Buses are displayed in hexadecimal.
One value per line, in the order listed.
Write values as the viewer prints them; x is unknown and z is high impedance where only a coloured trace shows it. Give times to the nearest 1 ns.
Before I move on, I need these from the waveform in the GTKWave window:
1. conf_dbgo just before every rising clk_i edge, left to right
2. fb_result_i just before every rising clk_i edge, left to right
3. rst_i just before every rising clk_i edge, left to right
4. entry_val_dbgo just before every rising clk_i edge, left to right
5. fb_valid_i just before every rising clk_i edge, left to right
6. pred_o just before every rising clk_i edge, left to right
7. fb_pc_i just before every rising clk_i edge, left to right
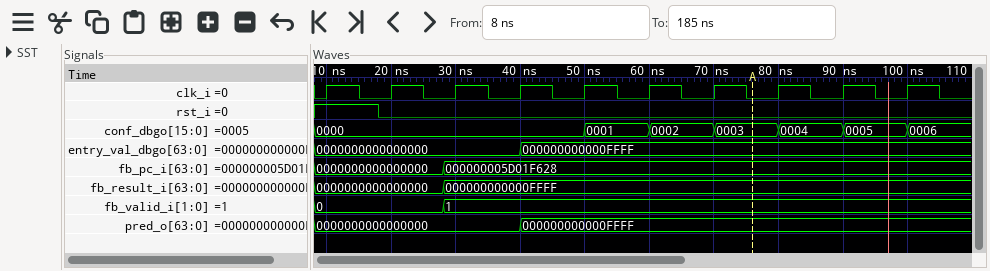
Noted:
0000, 0000, 0000, 0000, 0000, 0001, 0002, 0003, 0004, 0005
0000000000000000, 0000000000000000, 000000000000FFFF, 000000000000FFFF, 000000000000FFFF, 000000000000FFFF, 000000000000FFFF, 000000000000FFFF, 000000000000FFFF, 000000000000FFFF
1 0 0 0 0 0 0 0 0 0
0000000000000000, 0000000000000000, 0000000000000000, 0000000000000000, 000000000000FFFF, 000000000000FFFF, 000000000000FFFF, 000000000000FFFF, 000000000000FFFF, 000000000000FFFF
0, 0, 1, 1, 1, 1, 1, 1, 1, 1
0000000000000000, 0000000000000000, 0000000000000000, 0000000000000000, 000000000000FFFF, 000000000000FFFF, 000000000000FFFF, 000000000000FFFF, 000000000000FFFF, 000000000000FFFF
0000000000000000, 0000000000000000, 000000005D01F628, 000000005D01F628, 000000005D01F628, 000000005D01F628, 000000005D01F628, 000000005D01F628, 000000005D01F628, 000000005D01F628
